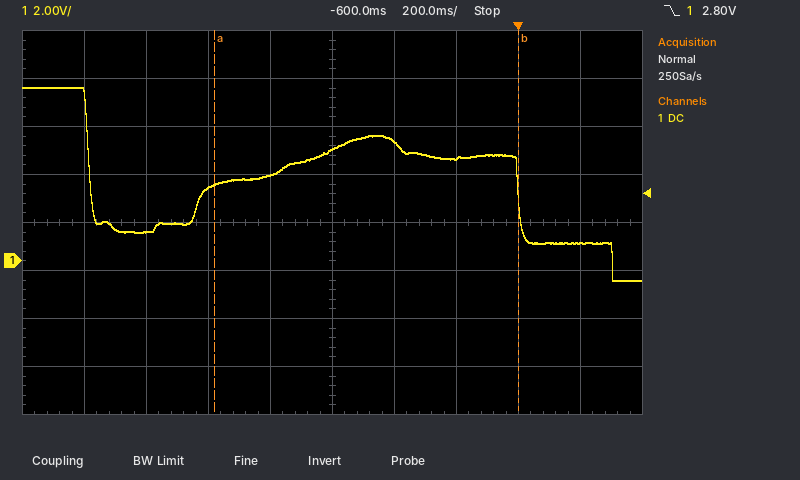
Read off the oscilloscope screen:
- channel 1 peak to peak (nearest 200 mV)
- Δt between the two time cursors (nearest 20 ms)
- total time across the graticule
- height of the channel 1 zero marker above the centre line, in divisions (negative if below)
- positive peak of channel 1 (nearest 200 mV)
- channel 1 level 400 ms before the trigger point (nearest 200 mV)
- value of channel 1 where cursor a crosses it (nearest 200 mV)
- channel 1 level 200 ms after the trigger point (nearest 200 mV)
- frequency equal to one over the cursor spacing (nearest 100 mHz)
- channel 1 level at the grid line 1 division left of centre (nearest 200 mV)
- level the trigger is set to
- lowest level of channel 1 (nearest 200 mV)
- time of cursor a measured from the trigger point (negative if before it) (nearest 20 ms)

8.0 V
980 ms
2 s
-0.8 div
7.2 V
5.0 V
3.2 V
800 mV
1.0 Hz
3.6 V
2.80 V
-800 mV
-980 ms
